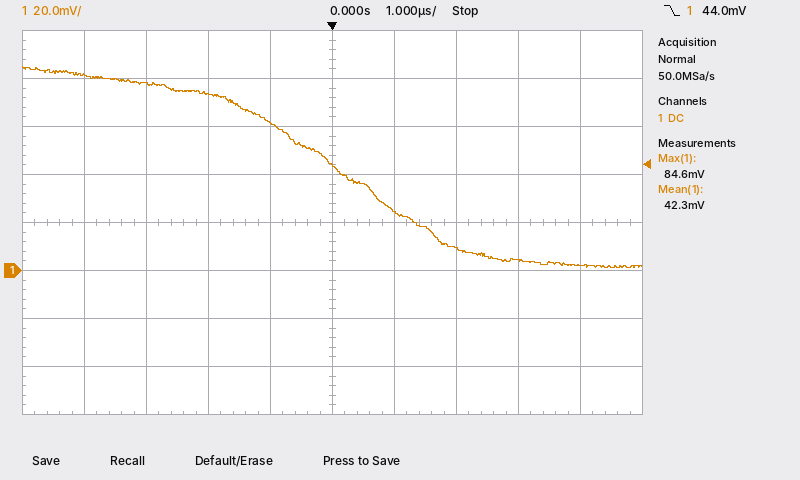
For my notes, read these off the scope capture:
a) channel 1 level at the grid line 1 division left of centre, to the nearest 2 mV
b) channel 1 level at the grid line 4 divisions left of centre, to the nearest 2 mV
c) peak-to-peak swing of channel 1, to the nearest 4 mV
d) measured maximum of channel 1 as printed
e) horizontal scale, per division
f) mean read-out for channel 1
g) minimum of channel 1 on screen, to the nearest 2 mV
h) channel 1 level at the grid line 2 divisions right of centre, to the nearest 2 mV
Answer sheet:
62 mV
82 mV
84 mV
84.6 mV
1 µs
42.3 mV
2 mV
10 mV
